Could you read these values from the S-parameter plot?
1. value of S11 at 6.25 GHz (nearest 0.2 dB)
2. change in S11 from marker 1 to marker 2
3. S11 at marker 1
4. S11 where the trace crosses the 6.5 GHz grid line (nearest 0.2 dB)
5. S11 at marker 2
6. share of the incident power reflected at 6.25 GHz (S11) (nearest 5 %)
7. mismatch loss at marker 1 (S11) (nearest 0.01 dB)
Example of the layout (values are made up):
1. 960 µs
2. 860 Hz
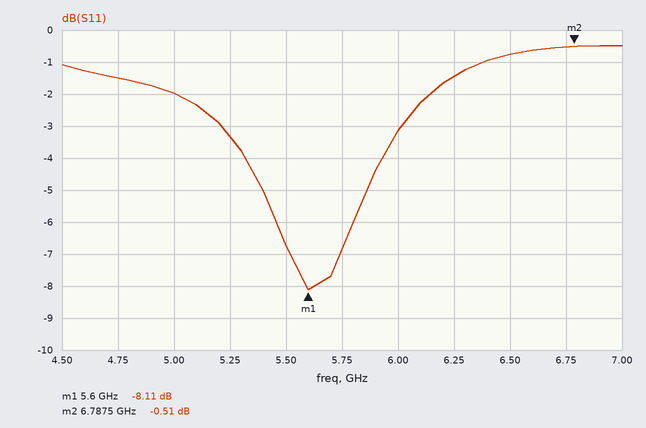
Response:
1. -1.4 dB
2. 7.60 dB
3. -8.11 dB
4. -0.8 dB
5. -0.51 dB
6. 70 %
7. 0.73 dB
